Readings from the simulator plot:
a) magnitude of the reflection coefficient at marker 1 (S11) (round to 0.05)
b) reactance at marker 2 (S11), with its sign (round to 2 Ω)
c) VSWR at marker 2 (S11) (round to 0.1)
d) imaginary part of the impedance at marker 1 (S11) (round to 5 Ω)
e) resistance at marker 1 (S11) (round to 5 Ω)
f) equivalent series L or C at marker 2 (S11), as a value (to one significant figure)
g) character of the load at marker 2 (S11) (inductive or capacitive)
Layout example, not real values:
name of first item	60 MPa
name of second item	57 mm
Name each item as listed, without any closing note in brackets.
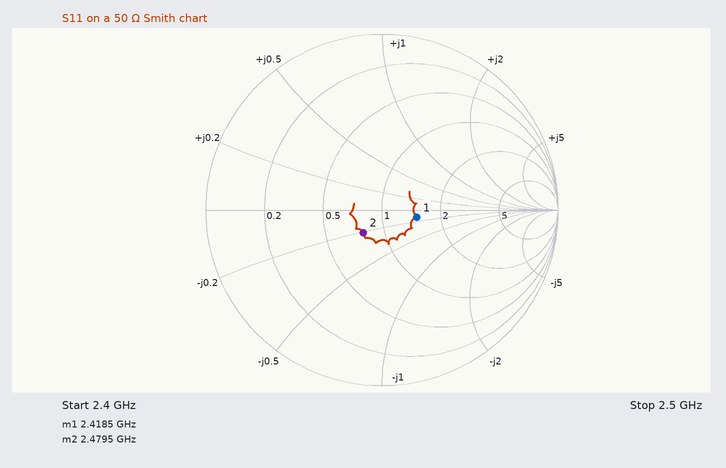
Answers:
magnitude of the reflection coefficient at marker 1 (S11)	0.20
reactance at marker 2 (S11), with its sign	-10 Ω
VSWR at marker 2 (S11)	1.4
imaginary part of the impedance at marker 1 (S11)	-5 Ω
resistance at marker 1 (S11)	75 Ω
equivalent series L or C at marker 2 (S11), as a value	6 pF
character of the load at marker 2 (S11)	capacitive
